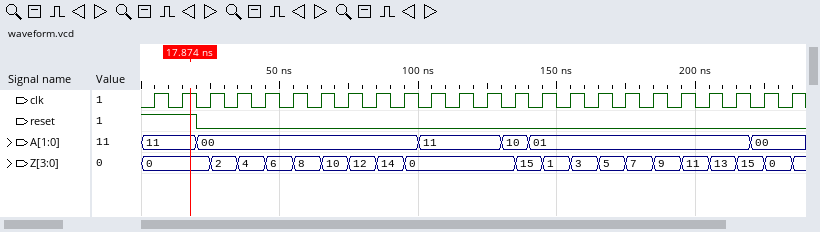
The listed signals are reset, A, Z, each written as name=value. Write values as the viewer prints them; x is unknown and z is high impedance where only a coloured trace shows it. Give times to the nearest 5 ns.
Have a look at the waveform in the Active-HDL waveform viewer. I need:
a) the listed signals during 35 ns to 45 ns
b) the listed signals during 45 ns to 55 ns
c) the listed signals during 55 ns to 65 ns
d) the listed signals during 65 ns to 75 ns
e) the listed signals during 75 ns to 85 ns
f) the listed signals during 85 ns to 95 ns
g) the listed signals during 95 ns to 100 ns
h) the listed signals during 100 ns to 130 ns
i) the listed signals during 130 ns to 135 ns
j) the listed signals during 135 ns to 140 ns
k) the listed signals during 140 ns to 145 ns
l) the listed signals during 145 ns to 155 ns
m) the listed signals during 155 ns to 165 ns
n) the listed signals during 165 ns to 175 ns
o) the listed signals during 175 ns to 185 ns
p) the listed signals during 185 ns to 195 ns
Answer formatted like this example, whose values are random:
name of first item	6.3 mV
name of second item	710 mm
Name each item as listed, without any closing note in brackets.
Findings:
the listed signals during 35 ns to 45 ns	reset=0, A=00, Z=4
the listed signals during 45 ns to 55 ns	reset=0, A=00, Z=6
the listed signals during 55 ns to 65 ns	reset=0, A=00, Z=8
the listed signals during 65 ns to 75 ns	reset=0, A=00, Z=10
the listed signals during 75 ns to 85 ns	reset=0, A=00, Z=12
the listed signals during 85 ns to 95 ns	reset=0, A=00, Z=14
the listed signals during 95 ns to 100 ns	reset=0, A=00, Z=0
the listed signals during 100 ns to 130 ns	reset=0, A=11, Z=0
the listed signals during 130 ns to 135 ns	reset=0, A=10, Z=0
the listed signals during 135 ns to 140 ns	reset=0, A=10, Z=15
the listed signals during 140 ns to 145 ns	reset=0, A=01, Z=15
the listed signals during 145 ns to 155 ns	reset=0, A=01, Z=1
the listed signals during 155 ns to 165 ns	reset=0, A=01, Z=3
the listed signals during 165 ns to 175 ns	reset=0, A=01, Z=5
the listed signals during 175 ns to 185 ns	reset=0, A=01, Z=7
the listed signals during 185 ns to 195 ns	reset=0, A=01, Z=9
